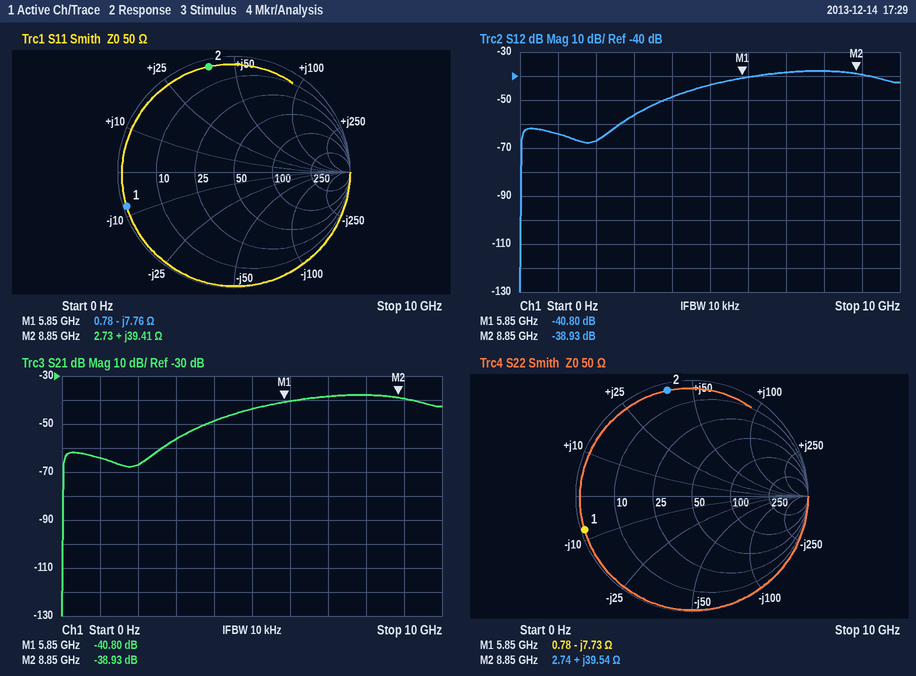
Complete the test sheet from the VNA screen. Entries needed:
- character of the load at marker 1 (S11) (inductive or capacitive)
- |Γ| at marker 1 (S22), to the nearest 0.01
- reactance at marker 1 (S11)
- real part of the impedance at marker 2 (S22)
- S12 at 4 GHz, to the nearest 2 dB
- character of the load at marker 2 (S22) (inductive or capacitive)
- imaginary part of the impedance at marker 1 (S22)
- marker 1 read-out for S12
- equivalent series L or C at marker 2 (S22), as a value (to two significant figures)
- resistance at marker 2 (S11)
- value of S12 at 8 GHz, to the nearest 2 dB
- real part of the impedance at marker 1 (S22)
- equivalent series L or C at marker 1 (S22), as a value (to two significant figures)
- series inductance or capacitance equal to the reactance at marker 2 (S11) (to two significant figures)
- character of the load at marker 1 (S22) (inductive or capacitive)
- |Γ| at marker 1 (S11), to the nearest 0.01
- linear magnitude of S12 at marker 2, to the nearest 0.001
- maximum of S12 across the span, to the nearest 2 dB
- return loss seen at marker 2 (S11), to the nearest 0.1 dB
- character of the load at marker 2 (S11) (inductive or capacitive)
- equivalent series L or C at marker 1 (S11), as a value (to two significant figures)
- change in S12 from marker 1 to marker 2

capacitive
0.97
-7.76 Ω
2.74 Ω
-48 dB
inductive
-7.73 Ω
-40.80 dB
710 pH
2.73 Ω
-38 dB
0.78 Ω
3.5 pF
710 pH
capacitive
0.97
0.011
-38 dB
0.6 dB
inductive
3.5 pF
1.87 dB
